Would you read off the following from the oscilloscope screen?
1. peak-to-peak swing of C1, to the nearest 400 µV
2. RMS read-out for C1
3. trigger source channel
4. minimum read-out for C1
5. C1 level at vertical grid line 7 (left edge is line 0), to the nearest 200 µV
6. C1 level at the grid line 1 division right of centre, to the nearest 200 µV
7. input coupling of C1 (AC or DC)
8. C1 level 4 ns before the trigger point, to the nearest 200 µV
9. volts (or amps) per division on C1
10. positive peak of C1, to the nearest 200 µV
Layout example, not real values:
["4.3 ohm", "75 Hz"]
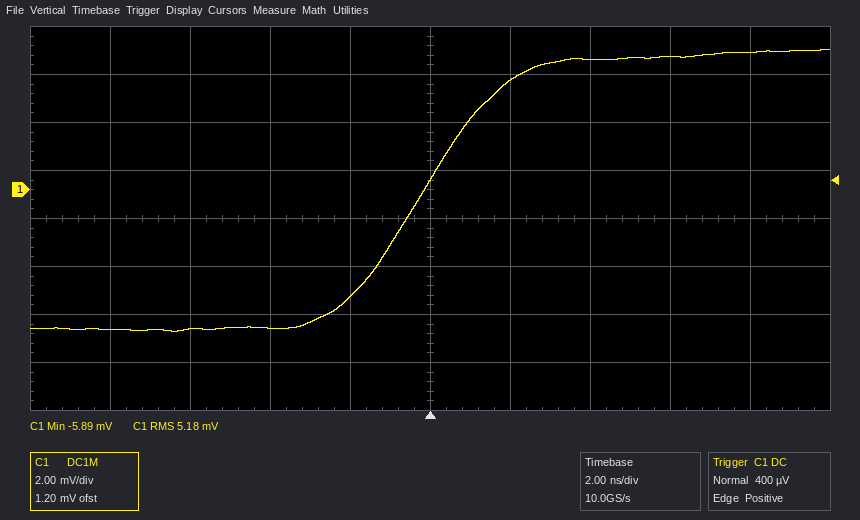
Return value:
["11.6 mV", "5.18 mV", "C1", "-5.89 mV", "5.4 mV", "4.6 mV", "DC", "-5.8 mV", "2 mV", "5.8 mV"]
